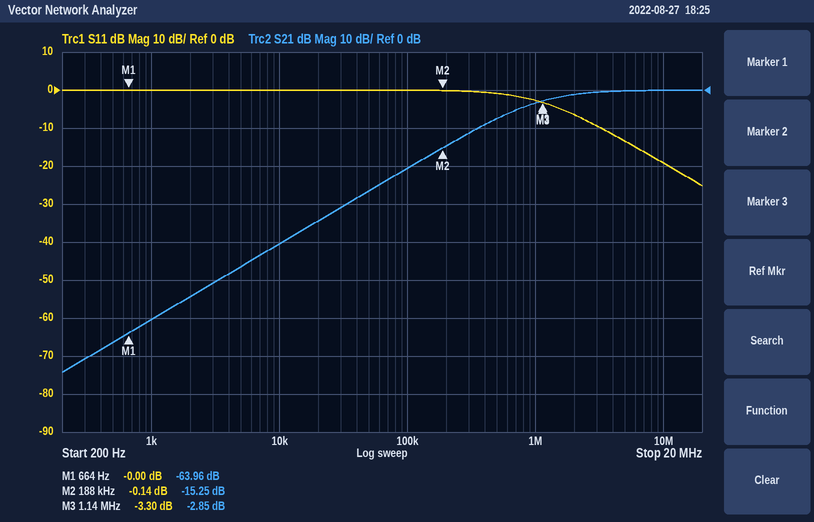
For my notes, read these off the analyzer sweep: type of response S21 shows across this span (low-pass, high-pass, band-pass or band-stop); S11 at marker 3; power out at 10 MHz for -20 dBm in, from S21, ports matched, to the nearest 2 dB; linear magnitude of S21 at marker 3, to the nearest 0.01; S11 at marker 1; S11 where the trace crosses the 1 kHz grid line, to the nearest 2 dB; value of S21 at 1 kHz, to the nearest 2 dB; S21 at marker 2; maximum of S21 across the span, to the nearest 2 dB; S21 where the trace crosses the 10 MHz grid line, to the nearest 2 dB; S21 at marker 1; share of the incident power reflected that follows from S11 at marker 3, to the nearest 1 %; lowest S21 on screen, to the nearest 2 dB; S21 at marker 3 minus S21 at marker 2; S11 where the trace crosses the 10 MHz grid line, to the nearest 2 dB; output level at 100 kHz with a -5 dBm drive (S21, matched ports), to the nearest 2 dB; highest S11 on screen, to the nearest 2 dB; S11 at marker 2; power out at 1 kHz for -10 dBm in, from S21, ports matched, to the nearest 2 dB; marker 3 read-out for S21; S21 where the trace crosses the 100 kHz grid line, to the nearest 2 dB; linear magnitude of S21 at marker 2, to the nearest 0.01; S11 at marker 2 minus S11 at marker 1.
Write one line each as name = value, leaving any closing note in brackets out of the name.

type of response S21 shows across this span = high-pass
S11 at marker 3 = -3.30 dB
power out at 10 MHz for -20 dBm in, from S21, ports matched, to the nearest 2 dB = -20 dBm
linear magnitude of S21 at marker 3, to the nearest 0.01 = 0.72
S11 at marker 1 = -0.00 dB
S11 where the trace crosses the 1 kHz grid line, to the nearest 2 dB = 0 dB
value of S21 at 1 kHz, to the nearest 2 dB = -60 dB
S21 at marker 2 = -15.25 dB
maximum of S21 across the span, to the nearest 2 dB = 0 dB
S21 where the trace crosses the 10 MHz grid line, to the nearest 2 dB = 0 dB
S21 at marker 1 = -63.96 dB
share of the incident power reflected that follows from S11 at marker 3, to the nearest 1 % = 47 %
lowest S21 on screen, to the nearest 2 dB = -74 dB
S21 at marker 3 minus S21 at marker 2 = 12.40 dB
S11 where the trace crosses the 10 MHz grid line, to the nearest 2 dB = -20 dB
output level at 100 kHz with a -5 dBm drive (S21, matched ports), to the nearest 2 dB = -26 dBm
highest S11 on screen, to the nearest 2 dB = 0 dB
S11 at marker 2 = -0.14 dB
power out at 1 kHz for -10 dBm in, from S21, ports matched, to the nearest 2 dB = -70 dBm
marker 3 read-out for S21 = -2.85 dB
S21 where the trace crosses the 100 kHz grid line, to the nearest 2 dB = -20 dB
linear magnitude of S21 at marker 2, to the nearest 0.01 = 0.17
S11 at marker 2 minus S11 at marker 1 = -0.14 dB
